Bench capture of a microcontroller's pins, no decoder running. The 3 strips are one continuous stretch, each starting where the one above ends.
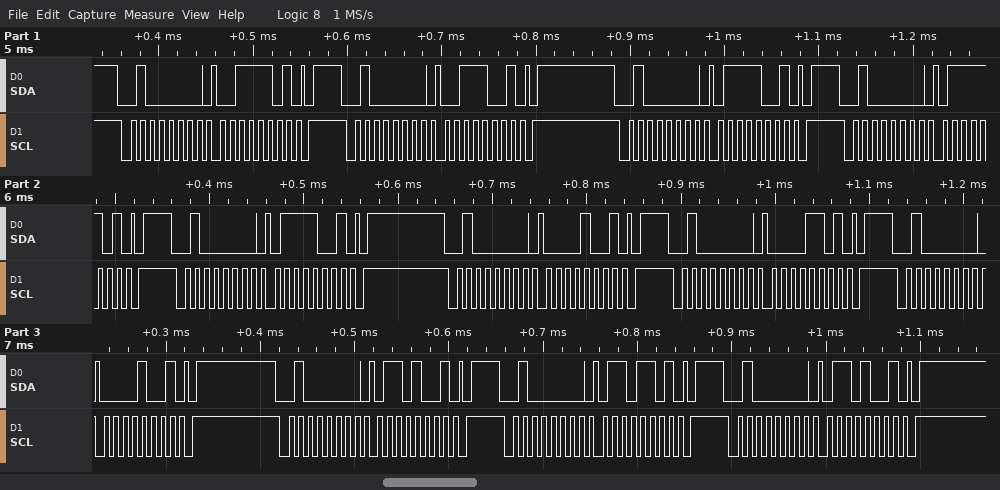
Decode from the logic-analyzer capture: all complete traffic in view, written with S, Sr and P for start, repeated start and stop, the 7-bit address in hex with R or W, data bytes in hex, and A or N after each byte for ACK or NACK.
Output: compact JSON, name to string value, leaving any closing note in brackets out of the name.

{"all complete traffic in view, written with S, Sr and P for start, repeated start and stop, the 7-bit address in hex with R or W, data bytes in hex, and A or N after each byte for ACK or NACK": "S 20W A 3D A P S 20W A 39 A P S 20W A 79 A P S 20W A 7D A P S 20W A 79 A P S 20W A 09 A P S 20W A 0D A P S 20W A 09 A P S 20W A 69 A P S 20W A 6D A P S 20W A 69 A P"}
